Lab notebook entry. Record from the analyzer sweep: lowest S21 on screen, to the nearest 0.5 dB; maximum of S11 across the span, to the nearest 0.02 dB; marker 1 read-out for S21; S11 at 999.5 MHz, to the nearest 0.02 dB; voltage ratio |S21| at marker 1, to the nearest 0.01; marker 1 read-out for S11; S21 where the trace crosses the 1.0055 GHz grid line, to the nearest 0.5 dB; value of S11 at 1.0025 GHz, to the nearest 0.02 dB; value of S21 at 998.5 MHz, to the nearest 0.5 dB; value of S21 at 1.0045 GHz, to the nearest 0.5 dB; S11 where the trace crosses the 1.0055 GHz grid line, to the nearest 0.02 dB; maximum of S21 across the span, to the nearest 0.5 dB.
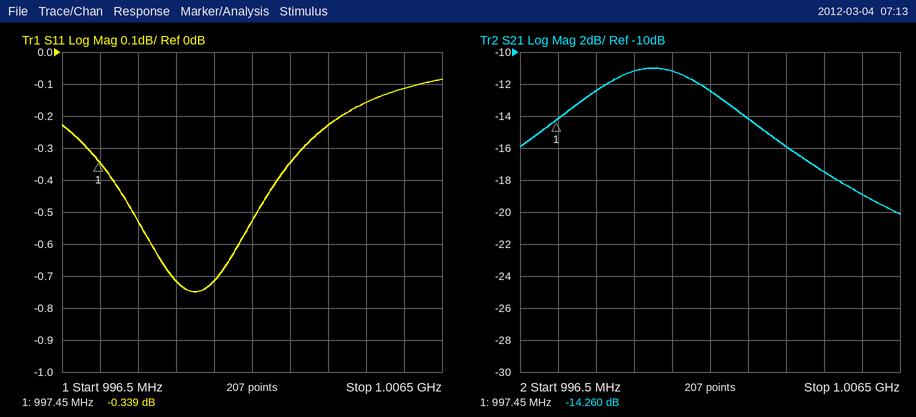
-20.0 dB
-0.08 dB
-14.260 dB
-0.72 dB
0.19
-0.339 dB
-19.0 dB
-0.34 dB
-12.5 dB
-17.5 dB
-0.12 dB
-11.0 dB
